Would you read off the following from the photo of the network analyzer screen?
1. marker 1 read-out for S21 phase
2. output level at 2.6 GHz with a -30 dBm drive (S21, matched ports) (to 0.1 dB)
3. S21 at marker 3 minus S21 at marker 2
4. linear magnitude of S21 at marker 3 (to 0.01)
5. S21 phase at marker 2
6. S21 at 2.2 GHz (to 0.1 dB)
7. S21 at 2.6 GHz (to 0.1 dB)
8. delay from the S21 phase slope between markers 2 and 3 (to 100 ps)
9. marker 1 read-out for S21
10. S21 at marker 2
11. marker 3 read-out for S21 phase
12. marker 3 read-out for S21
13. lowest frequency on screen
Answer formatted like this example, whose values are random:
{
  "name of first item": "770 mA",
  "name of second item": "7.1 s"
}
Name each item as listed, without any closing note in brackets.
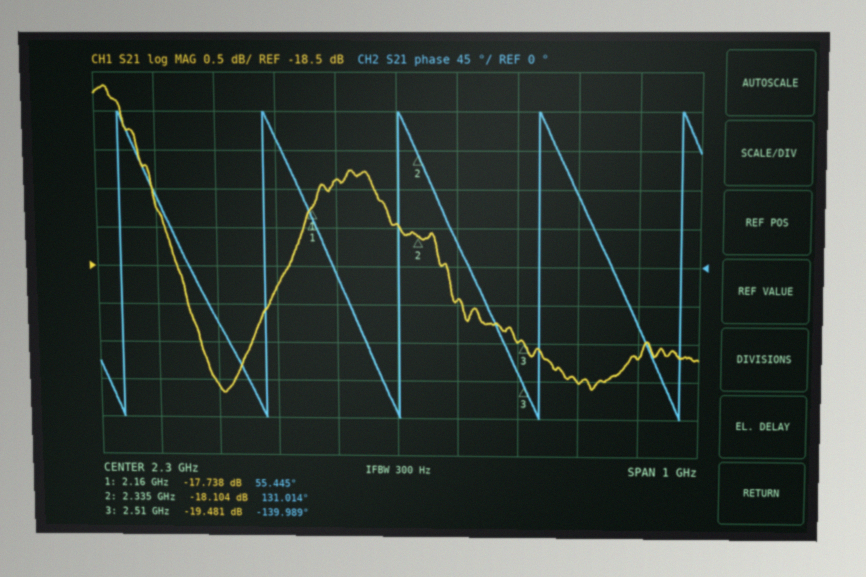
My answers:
{
  "marker 1 read-out for S21 phase": "55.445°",
  "output level at 2.6 GHz with a -30 dBm drive (S21, matched ports)": "-50.0 dBm",
  "S21 at marker 3 minus S21 at marker 2": "-1.377 dB",
  "linear magnitude of S21 at marker 3": "0.11",
  "S21 phase at marker 2": "131.014°",
  "S21 at 2.2 GHz": "-17.4 dB",
  "S21 at 2.6 GHz": "-20.0 dB",
  "delay from the S21 phase slope between markers 2 and 3": "4.3 ns",
  "marker 1 read-out for S21": "-17.738 dB",
  "S21 at marker 2": "-18.104 dB",
  "marker 3 read-out for S21 phase": "-139.989°",
  "marker 3 read-out for S21": "-19.481 dB",
  "lowest frequency on screen": "1.8 GHz"
}
